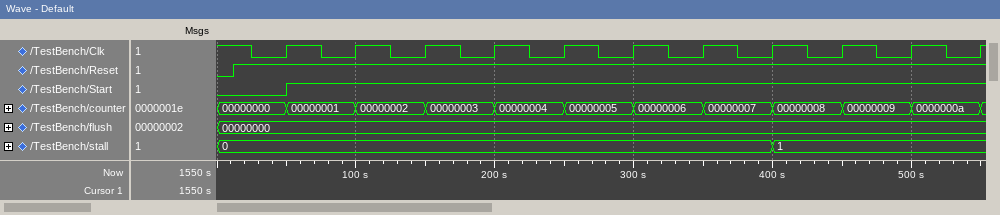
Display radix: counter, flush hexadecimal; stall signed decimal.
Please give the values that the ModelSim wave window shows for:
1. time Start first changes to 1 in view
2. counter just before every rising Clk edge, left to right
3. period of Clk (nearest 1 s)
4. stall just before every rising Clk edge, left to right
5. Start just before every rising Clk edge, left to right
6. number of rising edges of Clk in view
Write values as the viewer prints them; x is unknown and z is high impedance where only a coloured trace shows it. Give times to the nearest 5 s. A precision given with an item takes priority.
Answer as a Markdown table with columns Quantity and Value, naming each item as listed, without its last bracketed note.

| Quantity | Value |
|---|---|
| time Start first changes to 1 in view | 50 s |
| counter just before every rising Clk edge, left to right | 00000000, 00000001, 00000002, 00000003, 00000004, 00000005, 00000006, 00000007, 00000008, 00000009, 0000000a |
| period of Clk | 50 s |
| stall just before every rising Clk edge, left to right | 0, 0, 0, 0, 0, 0, 0, 0, 1, 1, 1 |
| Start just before every rising Clk edge, left to right | 0 1 1 1 1 1 1 1 1 1 1 |
| number of rising edges of Clk in view | 11 |
